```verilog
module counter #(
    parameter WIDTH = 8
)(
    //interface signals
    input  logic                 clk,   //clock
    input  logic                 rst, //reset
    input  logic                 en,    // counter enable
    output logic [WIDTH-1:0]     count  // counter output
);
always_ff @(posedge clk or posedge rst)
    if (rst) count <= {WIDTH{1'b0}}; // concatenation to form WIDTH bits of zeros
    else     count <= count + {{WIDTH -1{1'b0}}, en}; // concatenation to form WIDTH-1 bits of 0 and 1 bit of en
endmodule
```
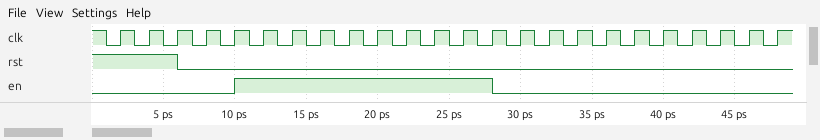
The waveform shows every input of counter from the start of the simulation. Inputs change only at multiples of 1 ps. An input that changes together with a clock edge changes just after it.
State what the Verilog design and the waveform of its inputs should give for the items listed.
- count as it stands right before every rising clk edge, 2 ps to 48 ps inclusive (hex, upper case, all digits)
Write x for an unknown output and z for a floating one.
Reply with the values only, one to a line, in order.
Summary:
00, 00, 00, 00, 00, 00, 01, 02, 03, 04, 05, 06, 07, 08, 09, 09, 09, 09, 09, 09, 09, 09, 09, 09
